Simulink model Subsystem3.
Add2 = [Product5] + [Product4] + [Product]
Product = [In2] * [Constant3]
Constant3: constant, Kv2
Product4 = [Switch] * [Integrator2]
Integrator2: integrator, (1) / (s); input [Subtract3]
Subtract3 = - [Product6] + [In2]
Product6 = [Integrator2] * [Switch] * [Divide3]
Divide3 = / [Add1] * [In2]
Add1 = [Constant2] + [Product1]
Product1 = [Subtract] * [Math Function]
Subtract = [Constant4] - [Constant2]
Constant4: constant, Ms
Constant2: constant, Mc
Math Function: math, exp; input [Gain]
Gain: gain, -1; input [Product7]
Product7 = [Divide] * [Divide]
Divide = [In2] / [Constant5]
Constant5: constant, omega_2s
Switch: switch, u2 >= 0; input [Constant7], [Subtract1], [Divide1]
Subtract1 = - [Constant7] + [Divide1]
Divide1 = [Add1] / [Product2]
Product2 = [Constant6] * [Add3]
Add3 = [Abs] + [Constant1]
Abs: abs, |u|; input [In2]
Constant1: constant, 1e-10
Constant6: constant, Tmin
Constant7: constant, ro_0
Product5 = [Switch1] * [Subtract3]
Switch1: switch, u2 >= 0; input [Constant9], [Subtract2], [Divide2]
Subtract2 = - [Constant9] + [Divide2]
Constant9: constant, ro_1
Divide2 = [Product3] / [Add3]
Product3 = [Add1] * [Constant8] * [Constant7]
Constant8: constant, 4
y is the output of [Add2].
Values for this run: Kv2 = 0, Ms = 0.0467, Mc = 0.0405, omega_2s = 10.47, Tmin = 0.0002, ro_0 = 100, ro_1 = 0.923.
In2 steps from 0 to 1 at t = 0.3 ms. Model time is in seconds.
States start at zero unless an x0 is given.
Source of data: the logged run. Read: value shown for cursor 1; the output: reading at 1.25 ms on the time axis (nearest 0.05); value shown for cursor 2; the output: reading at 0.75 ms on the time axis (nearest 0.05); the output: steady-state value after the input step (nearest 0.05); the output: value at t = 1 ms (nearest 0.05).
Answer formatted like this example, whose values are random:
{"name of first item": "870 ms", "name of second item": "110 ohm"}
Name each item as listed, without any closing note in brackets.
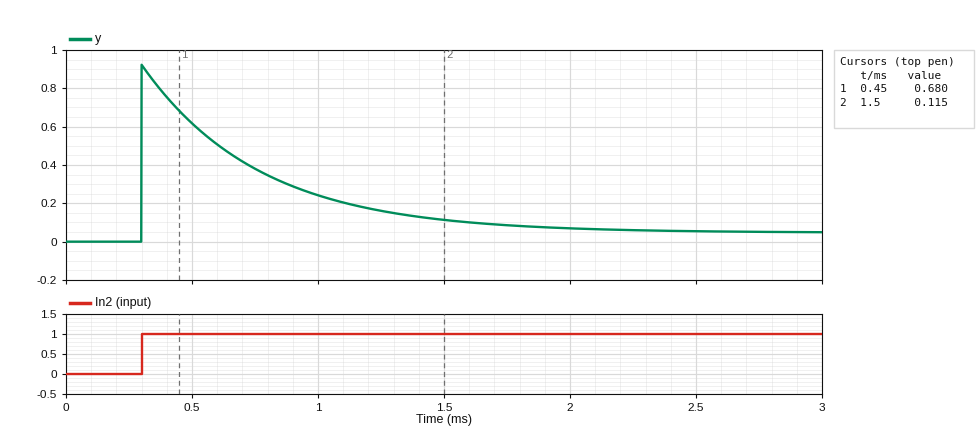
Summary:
{"value shown for cursor 1": "0.680", "the output: reading at 1.25 ms on the time axis": "0.15", "value shown for cursor 2": "0.115", "the output: reading at 0.75 ms on the time axis": "0.40", "the output: steady-state value after the input step": "0.05", "the output: value at t = 1 ms": "0.25"}
